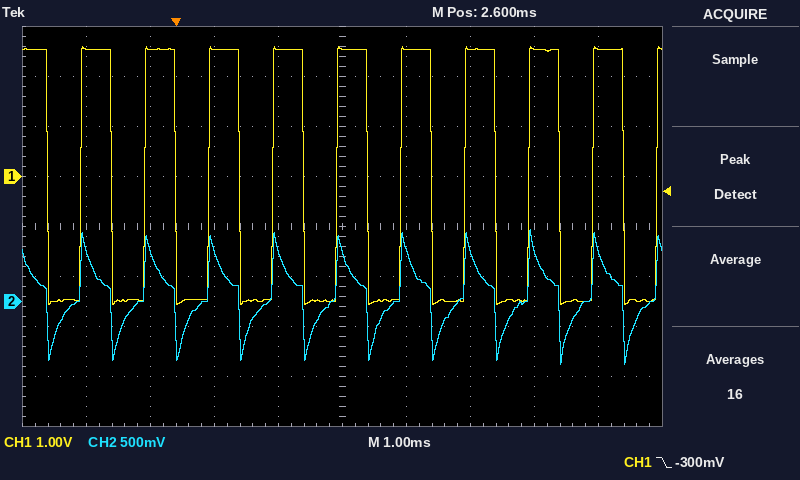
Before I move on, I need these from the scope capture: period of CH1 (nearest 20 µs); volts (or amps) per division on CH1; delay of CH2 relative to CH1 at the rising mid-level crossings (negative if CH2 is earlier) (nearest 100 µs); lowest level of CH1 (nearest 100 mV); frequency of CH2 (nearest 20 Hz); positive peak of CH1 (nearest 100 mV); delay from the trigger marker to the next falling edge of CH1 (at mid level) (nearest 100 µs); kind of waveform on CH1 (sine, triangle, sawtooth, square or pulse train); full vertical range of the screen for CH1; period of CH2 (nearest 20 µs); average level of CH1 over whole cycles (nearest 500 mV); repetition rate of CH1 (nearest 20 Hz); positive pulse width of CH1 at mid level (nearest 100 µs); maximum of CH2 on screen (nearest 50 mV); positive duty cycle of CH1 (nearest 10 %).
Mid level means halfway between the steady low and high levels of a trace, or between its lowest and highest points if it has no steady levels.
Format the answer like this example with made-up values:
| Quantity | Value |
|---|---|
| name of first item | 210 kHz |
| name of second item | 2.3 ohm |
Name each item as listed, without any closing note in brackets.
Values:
| Quantity | Value |
|---|---|
| period of CH1 | 1.00 ms |
| volts (or amps) per division on CH1 | 1 V |
| delay of CH2 relative to CH1 at the rising mid-level crossings (negative if CH2 is earlier) | 0.0 ms |
| lowest level of CH1 | -2.6 V |
| frequency of CH2 | 1.00 kHz |
| positive peak of CH1 | 2.6 V |
| delay from the trigger marker to the next falling edge of CH1 (at mid level) | 1.0 ms |
| kind of waveform on CH1 | square |
| full vertical range of the screen for CH1 | 8 V |
| period of CH2 | 1.00 ms |
| average level of CH1 over whole cycles | 0.0 V |
| repetition rate of CH1 | 1.00 kHz |
| positive pulse width of CH1 at mid level | 500 µs |
| maximum of CH2 on screen | 700 mV |
| positive duty cycle of CH1 | 50 % |
